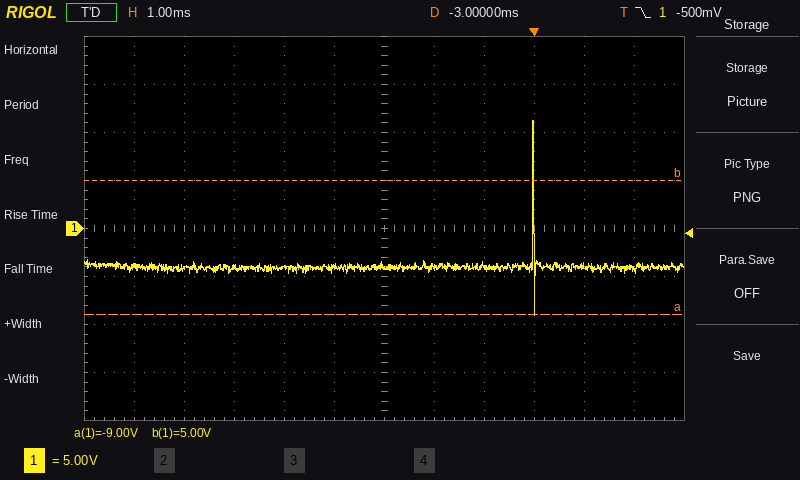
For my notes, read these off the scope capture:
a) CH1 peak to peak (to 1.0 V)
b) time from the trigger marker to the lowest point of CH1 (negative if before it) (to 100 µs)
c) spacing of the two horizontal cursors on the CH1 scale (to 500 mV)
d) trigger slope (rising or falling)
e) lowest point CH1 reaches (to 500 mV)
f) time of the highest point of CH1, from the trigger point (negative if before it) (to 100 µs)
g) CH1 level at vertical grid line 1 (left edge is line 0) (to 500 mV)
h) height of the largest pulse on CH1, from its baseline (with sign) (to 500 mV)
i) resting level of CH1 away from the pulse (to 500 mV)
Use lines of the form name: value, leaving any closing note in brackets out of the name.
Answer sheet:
CH1 peak to peak: 20.0 V
time from the trigger marker to the lowest point of CH1 (negative if before it): 0.0 ms
spacing of the two horizontal cursors on the CH1 scale: 14.0 V
trigger slope: falling
lowest point CH1 reaches: -9.0 V
time of the highest point of CH1, from the trigger point (negative if before it): 0.0 ms
CH1 level at vertical grid line 1 (left edge is line 0): -4.0 V
height of the largest pulse on CH1, from its baseline (with sign): +15.5 V
resting level of CH1 away from the pulse: -4.0 V
